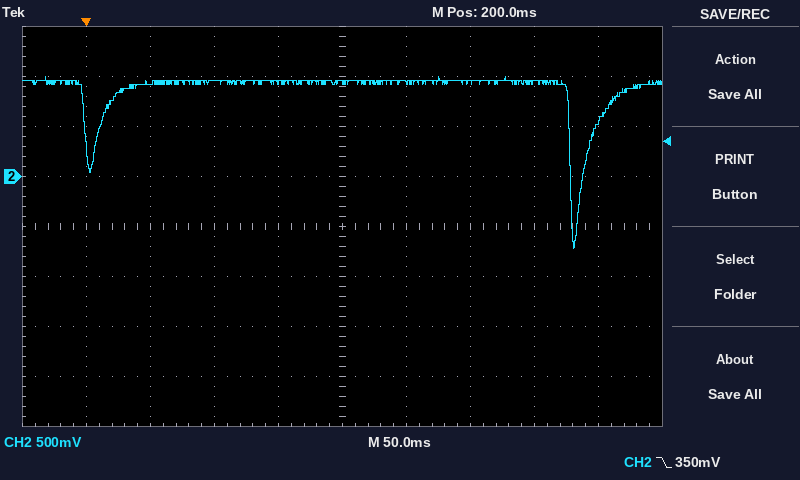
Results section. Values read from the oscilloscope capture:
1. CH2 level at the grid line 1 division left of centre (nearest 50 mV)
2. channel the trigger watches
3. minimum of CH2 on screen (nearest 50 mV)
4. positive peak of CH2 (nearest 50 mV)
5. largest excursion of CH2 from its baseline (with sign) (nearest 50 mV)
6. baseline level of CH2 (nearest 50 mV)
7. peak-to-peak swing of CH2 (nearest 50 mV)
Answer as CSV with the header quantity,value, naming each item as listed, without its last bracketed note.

quantity,value
CH2 level at the grid line 1 division left of centre,950 mV
channel the trigger watches,CH2
minimum of CH2 on screen,-700 mV
positive peak of CH2,1.00 V
largest excursion of CH2 from its baseline (with sign),-1.65 V
baseline level of CH2,950 mV
peak-to-peak swing of CH2,1.70 V
